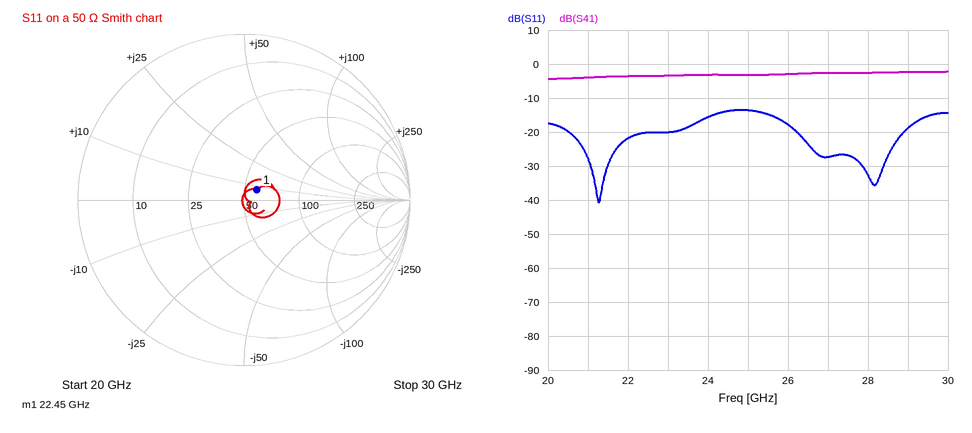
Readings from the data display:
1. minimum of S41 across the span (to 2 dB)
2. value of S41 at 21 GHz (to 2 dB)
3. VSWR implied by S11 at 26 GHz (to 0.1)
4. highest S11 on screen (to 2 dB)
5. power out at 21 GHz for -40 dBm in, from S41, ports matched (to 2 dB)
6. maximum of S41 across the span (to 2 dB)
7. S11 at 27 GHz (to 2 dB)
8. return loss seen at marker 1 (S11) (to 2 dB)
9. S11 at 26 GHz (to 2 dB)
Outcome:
-4 dB
-4 dB
1.3
-14 dB
-44 dBm
-2 dB
-28 dB
20 dB
-18 dB
